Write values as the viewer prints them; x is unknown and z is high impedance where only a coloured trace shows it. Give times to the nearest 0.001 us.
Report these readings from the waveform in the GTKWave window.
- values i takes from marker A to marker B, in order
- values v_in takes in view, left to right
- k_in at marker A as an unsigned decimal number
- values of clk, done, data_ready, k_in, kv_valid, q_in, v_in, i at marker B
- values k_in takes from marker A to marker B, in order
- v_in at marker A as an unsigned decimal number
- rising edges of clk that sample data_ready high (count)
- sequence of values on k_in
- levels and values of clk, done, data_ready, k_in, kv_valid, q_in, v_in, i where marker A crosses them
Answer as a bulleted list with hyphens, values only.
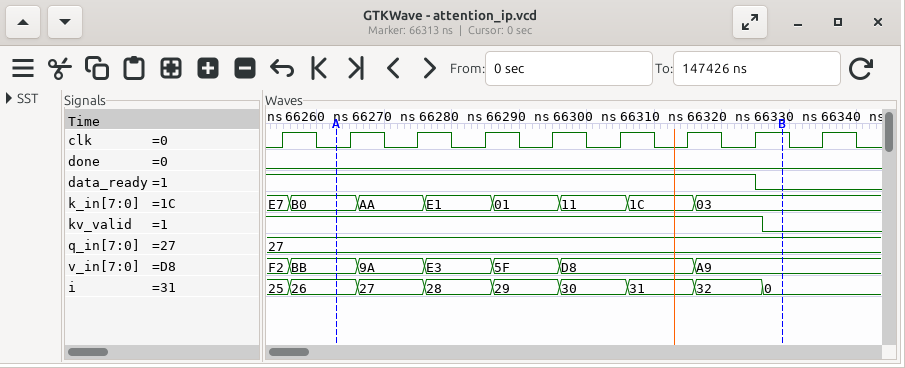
- 26, 27, 28, 29, 30, 31, 32, 0
- F2, BB, 9A, E3, 5F, D8, A9
- 176
- clk=1, done=0, data_ready=0, k_in=03, kv_valid=0, q_in=27, v_in=A9, i=0
- B0, AA, E1, 01, 11, 1C, 03
- 187
- 8
- E7, B0, AA, E1, 01, 11, 1C, 03
- clk=0, done=0, data_ready=1, k_in=B0, kv_valid=1, q_in=27, v_in=BB, i=26
